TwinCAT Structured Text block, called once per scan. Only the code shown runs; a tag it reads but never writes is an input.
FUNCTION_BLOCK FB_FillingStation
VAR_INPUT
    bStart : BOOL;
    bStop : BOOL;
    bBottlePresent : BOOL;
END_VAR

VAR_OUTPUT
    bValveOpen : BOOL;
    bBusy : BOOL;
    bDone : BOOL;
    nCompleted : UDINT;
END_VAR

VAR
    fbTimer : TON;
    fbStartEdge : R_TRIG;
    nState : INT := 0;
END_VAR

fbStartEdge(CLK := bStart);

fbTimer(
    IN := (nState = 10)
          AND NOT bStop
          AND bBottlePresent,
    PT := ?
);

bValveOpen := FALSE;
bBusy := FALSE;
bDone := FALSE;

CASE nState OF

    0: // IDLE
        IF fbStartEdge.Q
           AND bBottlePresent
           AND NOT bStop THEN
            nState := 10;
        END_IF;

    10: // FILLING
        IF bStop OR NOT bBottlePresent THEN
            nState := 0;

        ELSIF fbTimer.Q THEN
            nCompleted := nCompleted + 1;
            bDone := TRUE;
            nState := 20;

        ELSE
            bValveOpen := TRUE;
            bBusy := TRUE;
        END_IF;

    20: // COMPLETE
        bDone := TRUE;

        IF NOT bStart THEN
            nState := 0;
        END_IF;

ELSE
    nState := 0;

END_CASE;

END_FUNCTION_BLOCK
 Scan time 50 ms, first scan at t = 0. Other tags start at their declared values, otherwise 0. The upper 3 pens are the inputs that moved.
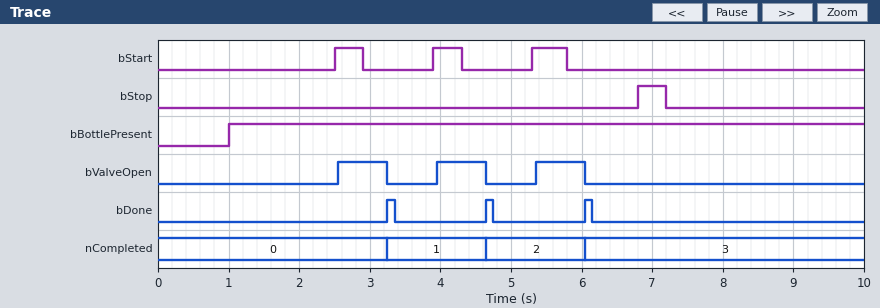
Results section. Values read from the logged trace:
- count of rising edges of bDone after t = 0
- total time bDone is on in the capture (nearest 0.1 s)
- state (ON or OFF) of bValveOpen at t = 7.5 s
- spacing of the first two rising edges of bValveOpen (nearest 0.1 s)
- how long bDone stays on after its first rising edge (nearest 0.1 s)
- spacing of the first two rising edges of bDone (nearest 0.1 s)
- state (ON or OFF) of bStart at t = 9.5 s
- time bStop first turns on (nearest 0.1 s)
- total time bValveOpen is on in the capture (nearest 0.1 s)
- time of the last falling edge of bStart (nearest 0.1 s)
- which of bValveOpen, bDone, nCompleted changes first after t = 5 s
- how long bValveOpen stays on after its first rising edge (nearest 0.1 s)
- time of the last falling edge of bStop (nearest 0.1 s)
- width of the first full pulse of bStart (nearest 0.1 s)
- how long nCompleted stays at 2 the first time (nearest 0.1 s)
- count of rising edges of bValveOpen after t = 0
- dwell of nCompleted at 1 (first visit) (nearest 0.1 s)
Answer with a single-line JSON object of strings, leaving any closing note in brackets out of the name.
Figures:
{"count of rising edges of bDone after t = 0": "3", "total time bDone is on in the capture": "0.3 s", "state (ON or OFF) of bValveOpen at t = 7.5 s": "OFF", "spacing of the first two rising edges of bValveOpen": "1.4 s", "how long bDone stays on after its first rising edge": "0.1 s", "spacing of the first two rising edges of bDone": "1.4 s", "state (ON or OFF) of bStart at t = 9.5 s": "OFF", "time bStop first turns on": "6.8 s", "total time bValveOpen is on in the capture": "2.1 s", "time of the last falling edge of bStart": "5.8 s", "which of bValveOpen, bDone, nCompleted changes first after t = 5 s": "bValveOpen", "how long bValveOpen stays on after its first rising edge": "0.7 s", "time of the last falling edge of bStop": "7.2 s", "width of the first full pulse of bStart": "0.4 s", "how long nCompleted stays at 2 the first time": "1.4 s", "count of rising edges of bValveOpen after t = 0": "3", "dwell of nCompleted at 1 (first visit)": "1.4 s"}
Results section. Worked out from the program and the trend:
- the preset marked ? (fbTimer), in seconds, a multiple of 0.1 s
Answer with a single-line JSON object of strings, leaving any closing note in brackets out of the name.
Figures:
{"the preset marked ? (fbTimer), in seconds, a multiple of 0.1 s": "0.7 s"}
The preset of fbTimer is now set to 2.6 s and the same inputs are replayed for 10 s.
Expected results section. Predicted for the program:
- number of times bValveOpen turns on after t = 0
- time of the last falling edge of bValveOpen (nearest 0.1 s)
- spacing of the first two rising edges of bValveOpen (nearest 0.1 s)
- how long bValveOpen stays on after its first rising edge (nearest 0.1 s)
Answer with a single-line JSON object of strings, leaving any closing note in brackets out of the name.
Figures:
{"number of times bValveOpen turns on after t = 0": "2", "time of the last falling edge of bValveOpen": "6.8 s", "spacing of the first two rising edges of bValveOpen": "2.8 s", "how long bValveOpen stays on after its first rising edge": "2.6 s"}
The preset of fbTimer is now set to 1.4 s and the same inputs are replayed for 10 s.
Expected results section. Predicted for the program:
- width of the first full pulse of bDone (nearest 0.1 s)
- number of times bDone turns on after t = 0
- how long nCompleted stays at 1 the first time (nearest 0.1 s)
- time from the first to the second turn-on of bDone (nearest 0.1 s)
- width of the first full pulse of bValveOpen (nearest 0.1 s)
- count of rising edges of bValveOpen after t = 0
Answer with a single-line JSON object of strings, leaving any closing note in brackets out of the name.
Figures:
{"width of the first full pulse of bDone": "0.4 s", "number of times bDone turns on after t = 0": "2", "how long nCompleted stays at 1 the first time": "2.8 s", "time from the first to the second turn-on of bDone": "2.8 s", "width of the first full pulse of bValveOpen": "1.4 s", "count of rising edges of bValveOpen after t = 0": "2"}
